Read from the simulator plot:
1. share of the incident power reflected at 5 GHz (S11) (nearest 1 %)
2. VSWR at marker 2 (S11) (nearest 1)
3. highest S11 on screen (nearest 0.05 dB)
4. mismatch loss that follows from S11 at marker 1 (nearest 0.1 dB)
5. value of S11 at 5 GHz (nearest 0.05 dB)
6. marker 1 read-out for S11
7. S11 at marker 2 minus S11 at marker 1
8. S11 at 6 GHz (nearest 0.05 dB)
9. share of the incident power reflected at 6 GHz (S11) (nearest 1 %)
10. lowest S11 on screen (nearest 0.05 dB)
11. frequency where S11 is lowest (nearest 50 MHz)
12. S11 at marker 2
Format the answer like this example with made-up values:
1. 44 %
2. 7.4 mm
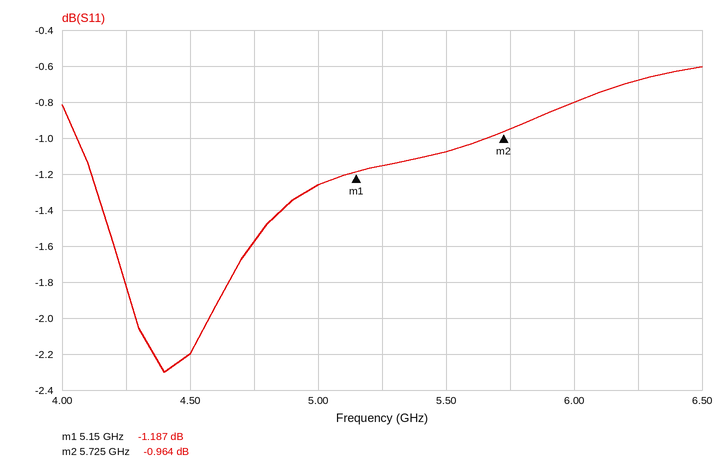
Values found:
1. 75 %
2. 18
3. -0.60 dB
4. 6.2 dB
5. -1.25 dB
6. -1.187 dB
7. 0.223 dB
8. -0.80 dB
9. 83 %
10. -2.30 dB
11. 4.40 GHz
12. -0.964 dB
